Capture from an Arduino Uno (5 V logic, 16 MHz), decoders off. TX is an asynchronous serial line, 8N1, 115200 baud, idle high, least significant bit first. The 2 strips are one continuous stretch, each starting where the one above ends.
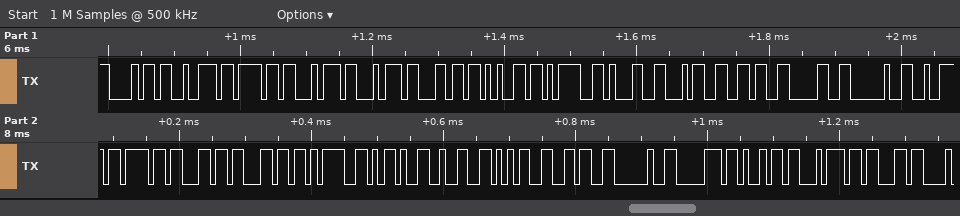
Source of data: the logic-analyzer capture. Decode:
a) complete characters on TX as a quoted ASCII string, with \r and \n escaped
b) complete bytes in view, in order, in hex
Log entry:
"hrottle=1460 roll=-256 pitc"
68 72 6F 74 74 6C 65 3D 31 34 36 30 20 72 6F 6C 6C 3D 2D 32 35 36 20 70 69 74 63
